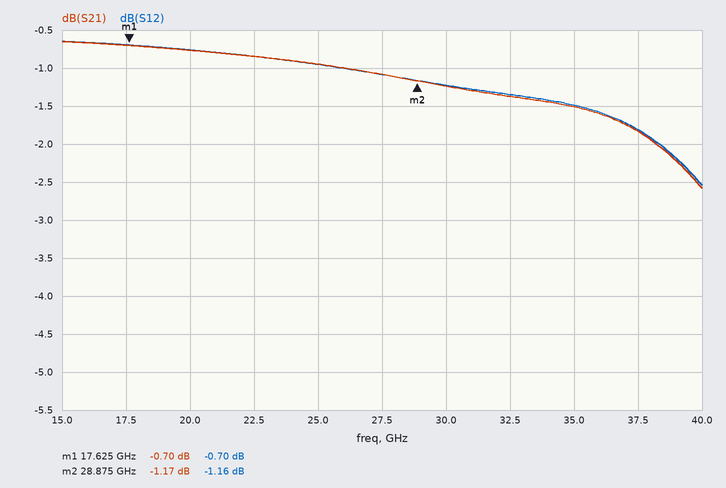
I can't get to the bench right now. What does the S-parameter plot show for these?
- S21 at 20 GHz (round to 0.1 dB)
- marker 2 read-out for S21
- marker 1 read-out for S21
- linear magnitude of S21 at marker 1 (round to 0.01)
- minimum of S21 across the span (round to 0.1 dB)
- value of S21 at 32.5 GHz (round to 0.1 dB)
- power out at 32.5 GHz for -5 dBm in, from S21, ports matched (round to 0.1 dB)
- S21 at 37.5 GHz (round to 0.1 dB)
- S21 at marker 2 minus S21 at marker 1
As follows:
-0.8 dB
-1.17 dB
-0.70 dB
0.92
-2.6 dB
-1.4 dB
-6.4 dBm
-1.8 dB
-0.47 dB
